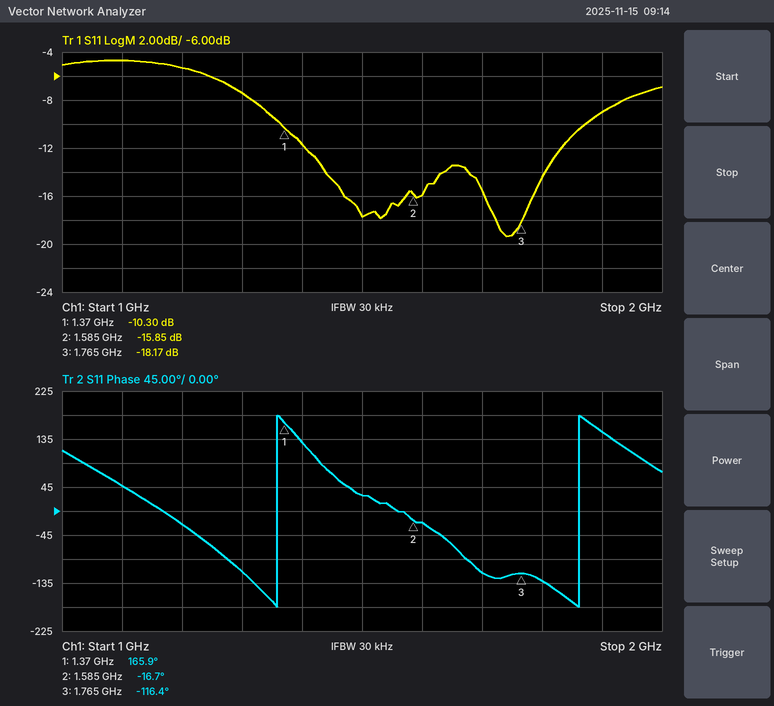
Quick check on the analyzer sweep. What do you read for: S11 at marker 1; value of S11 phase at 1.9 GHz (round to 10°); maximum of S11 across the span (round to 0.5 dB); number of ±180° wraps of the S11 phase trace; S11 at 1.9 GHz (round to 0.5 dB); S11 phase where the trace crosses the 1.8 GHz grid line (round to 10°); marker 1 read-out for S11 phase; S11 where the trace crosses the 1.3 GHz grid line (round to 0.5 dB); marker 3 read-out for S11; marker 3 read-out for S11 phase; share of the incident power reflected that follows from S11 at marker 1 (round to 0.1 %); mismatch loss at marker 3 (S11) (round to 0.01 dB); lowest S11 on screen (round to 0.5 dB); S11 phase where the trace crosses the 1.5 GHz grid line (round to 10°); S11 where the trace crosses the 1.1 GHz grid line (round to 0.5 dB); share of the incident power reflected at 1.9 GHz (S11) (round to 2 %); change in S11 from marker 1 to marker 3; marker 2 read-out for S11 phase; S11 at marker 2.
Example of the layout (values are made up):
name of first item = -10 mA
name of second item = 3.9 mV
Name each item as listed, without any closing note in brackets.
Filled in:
S11 at marker 1 = -10.30 dB
value of S11 phase at 1.9 GHz = 150°
maximum of S11 across the span = -4.5 dB
number of ±180° wraps of the S11 phase trace = 2
S11 at 1.9 GHz = -9.0 dB
S11 phase where the trace crosses the 1.8 GHz grid line = -130°
marker 1 read-out for S11 phase = 165.9°
S11 where the trace crosses the 1.3 GHz grid line = -7.5 dB
marker 3 read-out for S11 = -18.17 dB
marker 3 read-out for S11 phase = -116.4°
share of the incident power reflected that follows from S11 at marker 1 = 9.3 %
mismatch loss at marker 3 (S11) = 0.07 dB
lowest S11 on screen = -19.5 dB
S11 phase where the trace crosses the 1.5 GHz grid line = 30°
S11 where the trace crosses the 1.1 GHz grid line = -4.5 dB
share of the incident power reflected at 1.9 GHz (S11) = 12 %
change in S11 from marker 1 to marker 3 = -7.87 dB
marker 2 read-out for S11 phase = -16.7°
S11 at marker 2 = -15.85 dB
